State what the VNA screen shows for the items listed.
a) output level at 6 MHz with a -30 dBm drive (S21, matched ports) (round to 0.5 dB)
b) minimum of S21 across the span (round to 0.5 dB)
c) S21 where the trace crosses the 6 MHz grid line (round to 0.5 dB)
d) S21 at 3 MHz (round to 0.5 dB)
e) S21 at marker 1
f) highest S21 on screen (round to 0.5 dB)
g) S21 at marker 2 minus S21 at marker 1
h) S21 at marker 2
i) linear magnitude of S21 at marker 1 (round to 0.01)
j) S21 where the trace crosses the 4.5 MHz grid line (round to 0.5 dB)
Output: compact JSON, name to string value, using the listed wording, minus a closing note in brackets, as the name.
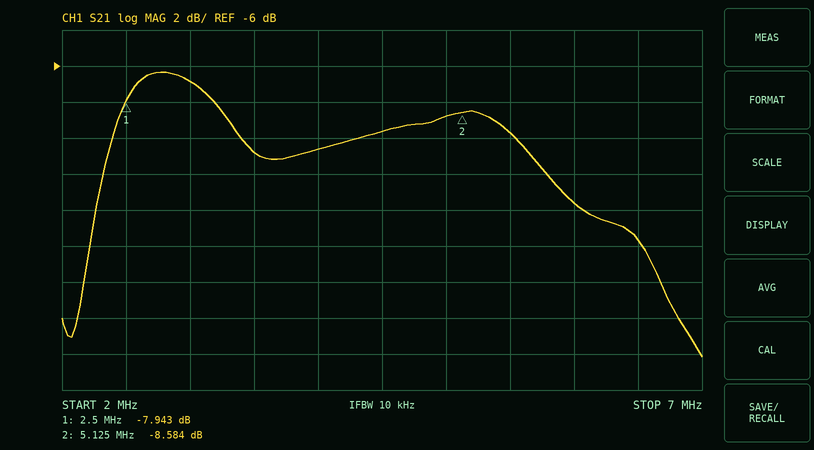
{"output level at 6 MHz with a -30 dBm drive (S21, matched ports)": "-43.5 dBm", "minimum of S21 across the span": "-22.0 dB", "S21 where the trace crosses the 6 MHz grid line": "-13.5 dB", "S21 at 3 MHz": "-7.0 dB", "S21 at marker 1": "-7.943 dB", "highest S21 on screen": "-6.5 dB", "S21 at marker 2 minus S21 at marker 1": "-0.641 dB", "S21 at marker 2": "-8.584 dB", "linear magnitude of S21 at marker 1": "0.40", "S21 where the trace crosses the 4.5 MHz grid line": "-9.5 dB"}
